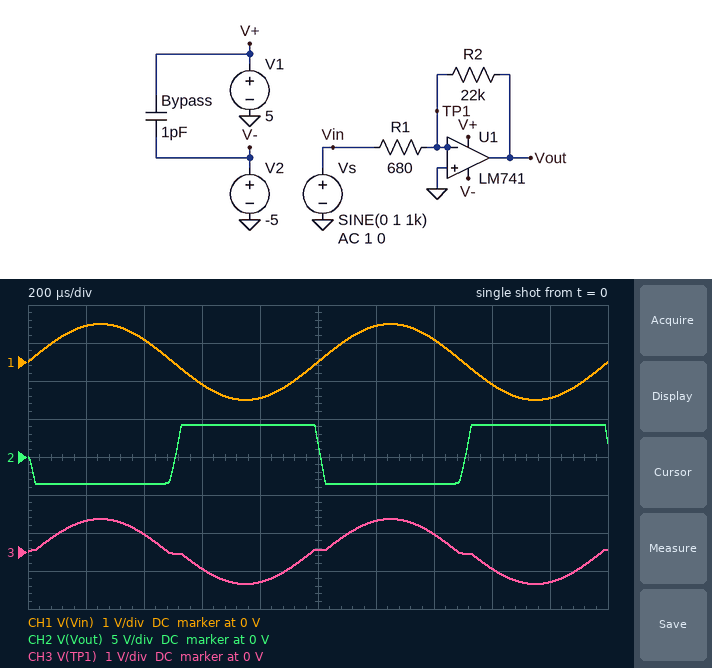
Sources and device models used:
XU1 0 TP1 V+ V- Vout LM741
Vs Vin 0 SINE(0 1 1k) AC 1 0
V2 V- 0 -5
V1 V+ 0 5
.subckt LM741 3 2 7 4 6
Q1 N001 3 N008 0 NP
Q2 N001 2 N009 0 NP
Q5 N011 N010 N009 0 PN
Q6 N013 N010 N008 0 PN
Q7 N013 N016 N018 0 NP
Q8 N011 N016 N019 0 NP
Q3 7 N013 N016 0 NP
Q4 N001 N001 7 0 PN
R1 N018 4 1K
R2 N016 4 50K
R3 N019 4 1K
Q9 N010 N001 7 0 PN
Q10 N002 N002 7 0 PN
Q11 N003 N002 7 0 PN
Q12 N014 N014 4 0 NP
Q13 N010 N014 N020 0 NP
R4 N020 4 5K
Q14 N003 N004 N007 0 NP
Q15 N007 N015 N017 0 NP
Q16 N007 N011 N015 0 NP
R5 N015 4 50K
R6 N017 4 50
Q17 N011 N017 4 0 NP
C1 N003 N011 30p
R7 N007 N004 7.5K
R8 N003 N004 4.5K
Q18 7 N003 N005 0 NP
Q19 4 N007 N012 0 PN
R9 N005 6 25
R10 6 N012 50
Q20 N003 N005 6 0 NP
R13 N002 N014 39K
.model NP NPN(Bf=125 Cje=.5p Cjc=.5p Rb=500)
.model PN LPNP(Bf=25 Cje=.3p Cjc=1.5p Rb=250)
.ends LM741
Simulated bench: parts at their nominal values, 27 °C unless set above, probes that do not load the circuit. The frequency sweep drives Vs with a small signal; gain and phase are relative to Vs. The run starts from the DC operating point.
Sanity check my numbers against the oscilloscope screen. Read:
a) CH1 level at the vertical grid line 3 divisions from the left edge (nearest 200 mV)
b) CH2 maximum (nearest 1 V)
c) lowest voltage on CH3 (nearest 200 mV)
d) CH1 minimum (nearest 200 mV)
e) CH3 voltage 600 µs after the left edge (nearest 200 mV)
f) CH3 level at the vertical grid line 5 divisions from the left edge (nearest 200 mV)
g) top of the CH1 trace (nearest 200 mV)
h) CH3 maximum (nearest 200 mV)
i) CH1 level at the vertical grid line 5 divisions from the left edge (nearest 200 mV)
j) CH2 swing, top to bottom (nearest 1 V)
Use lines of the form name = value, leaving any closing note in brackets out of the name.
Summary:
CH1 level at the vertical grid line 3 divisions from the left edge = -600 mV
CH2 maximum = 4 V
lowest voltage on CH3 = -800 mV
CH1 minimum = -1.0 V
CH3 voltage 600 µs after the left edge = -400 mV
CH3 level at the vertical grid line 5 divisions from the left edge = 0 V
top of the CH1 trace = 1.0 V
CH3 maximum = 800 mV
CH1 level at the vertical grid line 5 divisions from the left edge = 0 V
CH2 swing, top to bottom = 8 V
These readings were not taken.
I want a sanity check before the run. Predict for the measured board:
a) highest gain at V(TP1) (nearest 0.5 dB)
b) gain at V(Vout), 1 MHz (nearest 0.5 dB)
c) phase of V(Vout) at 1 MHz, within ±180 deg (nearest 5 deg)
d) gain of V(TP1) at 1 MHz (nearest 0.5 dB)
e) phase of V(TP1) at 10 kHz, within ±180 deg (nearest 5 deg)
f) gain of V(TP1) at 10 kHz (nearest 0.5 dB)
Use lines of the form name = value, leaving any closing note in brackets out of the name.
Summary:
highest gain at V(TP1) = 0 dB
gain at V(Vout), 1 MHz = -5.0 dB
phase of V(Vout) at 1 MHz, within ±180 deg = 30 deg
gain of V(TP1) at 1 MHz = 0 dB
phase of V(TP1) at 10 kHz, within ±180 deg = 45 deg
gain of V(TP1) at 10 kHz = -3.0 dB
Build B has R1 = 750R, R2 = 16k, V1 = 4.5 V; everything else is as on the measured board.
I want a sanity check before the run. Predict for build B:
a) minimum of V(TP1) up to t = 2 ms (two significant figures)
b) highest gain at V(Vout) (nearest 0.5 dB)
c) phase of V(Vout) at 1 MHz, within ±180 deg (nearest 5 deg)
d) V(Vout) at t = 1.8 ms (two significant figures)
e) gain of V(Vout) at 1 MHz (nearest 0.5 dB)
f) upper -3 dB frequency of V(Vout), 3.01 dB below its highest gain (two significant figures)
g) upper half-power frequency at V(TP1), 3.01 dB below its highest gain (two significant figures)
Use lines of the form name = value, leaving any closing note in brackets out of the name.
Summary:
minimum of V(TP1) up to t = 2 ms = -790 mV
highest gain at V(Vout) = 26.5 dB
phase of V(Vout) at 1 MHz, within ±180 deg = 20 deg
V(Vout) at t = 1.8 ms = 3.7 V
gain of V(Vout) at 1 MHz = -4.0 dB
upper -3 dB frequency of V(Vout), 3.01 dB below its highest gain = 12 kHz
upper half-power frequency at V(TP1), 3.01 dB below its highest gain = 300 MHz
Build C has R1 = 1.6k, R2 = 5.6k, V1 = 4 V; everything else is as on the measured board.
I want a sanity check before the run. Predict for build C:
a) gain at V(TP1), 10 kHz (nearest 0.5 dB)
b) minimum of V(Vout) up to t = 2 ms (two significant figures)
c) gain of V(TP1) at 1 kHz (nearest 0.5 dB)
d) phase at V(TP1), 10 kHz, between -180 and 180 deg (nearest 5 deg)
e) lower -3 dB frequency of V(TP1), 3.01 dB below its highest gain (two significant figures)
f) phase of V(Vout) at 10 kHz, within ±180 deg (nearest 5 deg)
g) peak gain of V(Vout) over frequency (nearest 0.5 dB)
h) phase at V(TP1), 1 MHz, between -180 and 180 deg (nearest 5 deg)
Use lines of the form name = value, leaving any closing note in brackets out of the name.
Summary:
gain at V(TP1), 10 kHz = -9.5 dB
minimum of V(Vout) up to t = 2 ms = -3.4 V
gain of V(TP1) at 1 kHz = -29.0 dB
phase at V(TP1), 10 kHz, between -180 and 180 deg = 70 deg
lower -3 dB frequency of V(TP1), 3.01 dB below its highest gain = 27 kHz
phase of V(Vout) at 10 kHz, within ±180 deg = 155 deg
peak gain of V(Vout) over frequency = 11.0 dB
phase at V(TP1), 1 MHz, between -180 and 180 deg = 0 deg
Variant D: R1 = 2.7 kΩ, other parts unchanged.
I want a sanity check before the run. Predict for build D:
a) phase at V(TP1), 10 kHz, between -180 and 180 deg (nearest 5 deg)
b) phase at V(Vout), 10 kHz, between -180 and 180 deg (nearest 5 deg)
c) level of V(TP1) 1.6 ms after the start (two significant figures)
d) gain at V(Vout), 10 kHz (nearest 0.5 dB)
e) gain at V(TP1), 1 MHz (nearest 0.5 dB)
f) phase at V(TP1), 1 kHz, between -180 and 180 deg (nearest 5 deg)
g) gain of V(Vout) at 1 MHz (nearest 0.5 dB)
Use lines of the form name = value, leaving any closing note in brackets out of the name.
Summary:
phase at V(TP1), 10 kHz, between -180 and 180 deg = 75 deg
phase at V(Vout), 10 kHz, between -180 and 180 deg = 165 deg
level of V(TP1) 1.6 ms after the start = -60 mV
gain at V(Vout), 10 kHz = 18.0 dB
gain at V(TP1), 1 MHz = -0.5 dB
phase at V(TP1), 1 kHz, between -180 and 180 deg = 90 deg
gain of V(Vout) at 1 MHz = -5.5 dB
